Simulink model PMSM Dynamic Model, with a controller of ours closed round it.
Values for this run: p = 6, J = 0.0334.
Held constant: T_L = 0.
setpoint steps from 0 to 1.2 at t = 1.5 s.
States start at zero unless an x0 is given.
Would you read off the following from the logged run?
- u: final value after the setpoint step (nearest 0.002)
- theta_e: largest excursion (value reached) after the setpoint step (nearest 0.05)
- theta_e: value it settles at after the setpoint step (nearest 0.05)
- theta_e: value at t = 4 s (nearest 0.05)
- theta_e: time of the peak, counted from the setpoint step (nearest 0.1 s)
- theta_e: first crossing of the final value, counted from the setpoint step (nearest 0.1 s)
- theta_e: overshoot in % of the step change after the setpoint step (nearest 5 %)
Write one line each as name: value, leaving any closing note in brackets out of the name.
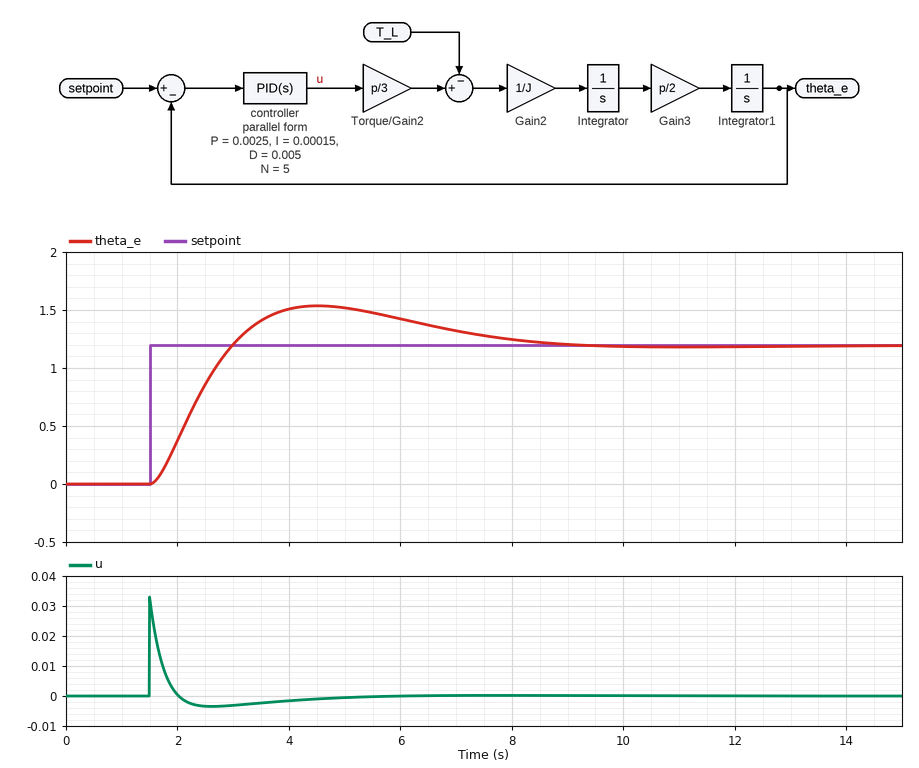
u: final value after the setpoint step: 0.000
theta_e: largest excursion (value reached) after the setpoint step: 1.55
theta_e: value it settles at after the setpoint step: 1.20
theta_e: value at t = 4 s: 1.50
theta_e: time of the peak, counted from the setpoint step: 3.0 s
theta_e: first crossing of the final value, counted from the setpoint step: 1.5 s
theta_e: overshoot in % of the step change after the setpoint step: 30 %
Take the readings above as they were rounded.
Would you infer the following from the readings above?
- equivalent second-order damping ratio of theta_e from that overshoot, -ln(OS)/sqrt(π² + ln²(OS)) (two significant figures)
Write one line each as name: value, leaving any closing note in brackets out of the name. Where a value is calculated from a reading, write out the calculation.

equivalent second-order damping ratio of theta_e from that overshoot, -ln(OS)/sqrt(π² + ln²(OS)): ln(0.3) = -1.204; 1.204 / sqrt(9.870 + 1.450) = 0.36
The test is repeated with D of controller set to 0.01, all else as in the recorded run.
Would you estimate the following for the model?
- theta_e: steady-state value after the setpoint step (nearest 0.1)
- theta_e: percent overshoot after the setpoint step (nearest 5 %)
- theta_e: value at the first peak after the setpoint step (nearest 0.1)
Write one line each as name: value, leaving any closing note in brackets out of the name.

theta_e: steady-state value after the setpoint step: 1.2
theta_e: percent overshoot after the setpoint step: 15 %
theta_e: value at the first peak after the setpoint step: 1.4
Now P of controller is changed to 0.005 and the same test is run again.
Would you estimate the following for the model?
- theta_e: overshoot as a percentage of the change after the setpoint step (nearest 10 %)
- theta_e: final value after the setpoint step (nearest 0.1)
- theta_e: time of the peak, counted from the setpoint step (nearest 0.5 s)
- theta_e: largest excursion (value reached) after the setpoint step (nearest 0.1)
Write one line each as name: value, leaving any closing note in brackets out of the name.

theta_e: overshoot as a percentage of the change after the setpoint step: 40 %
theta_e: final value after the setpoint step: 1.2
theta_e: time of the peak, counted from the setpoint step: 2.5 s
theta_e: largest excursion (value reached) after the setpoint step: 1.7
